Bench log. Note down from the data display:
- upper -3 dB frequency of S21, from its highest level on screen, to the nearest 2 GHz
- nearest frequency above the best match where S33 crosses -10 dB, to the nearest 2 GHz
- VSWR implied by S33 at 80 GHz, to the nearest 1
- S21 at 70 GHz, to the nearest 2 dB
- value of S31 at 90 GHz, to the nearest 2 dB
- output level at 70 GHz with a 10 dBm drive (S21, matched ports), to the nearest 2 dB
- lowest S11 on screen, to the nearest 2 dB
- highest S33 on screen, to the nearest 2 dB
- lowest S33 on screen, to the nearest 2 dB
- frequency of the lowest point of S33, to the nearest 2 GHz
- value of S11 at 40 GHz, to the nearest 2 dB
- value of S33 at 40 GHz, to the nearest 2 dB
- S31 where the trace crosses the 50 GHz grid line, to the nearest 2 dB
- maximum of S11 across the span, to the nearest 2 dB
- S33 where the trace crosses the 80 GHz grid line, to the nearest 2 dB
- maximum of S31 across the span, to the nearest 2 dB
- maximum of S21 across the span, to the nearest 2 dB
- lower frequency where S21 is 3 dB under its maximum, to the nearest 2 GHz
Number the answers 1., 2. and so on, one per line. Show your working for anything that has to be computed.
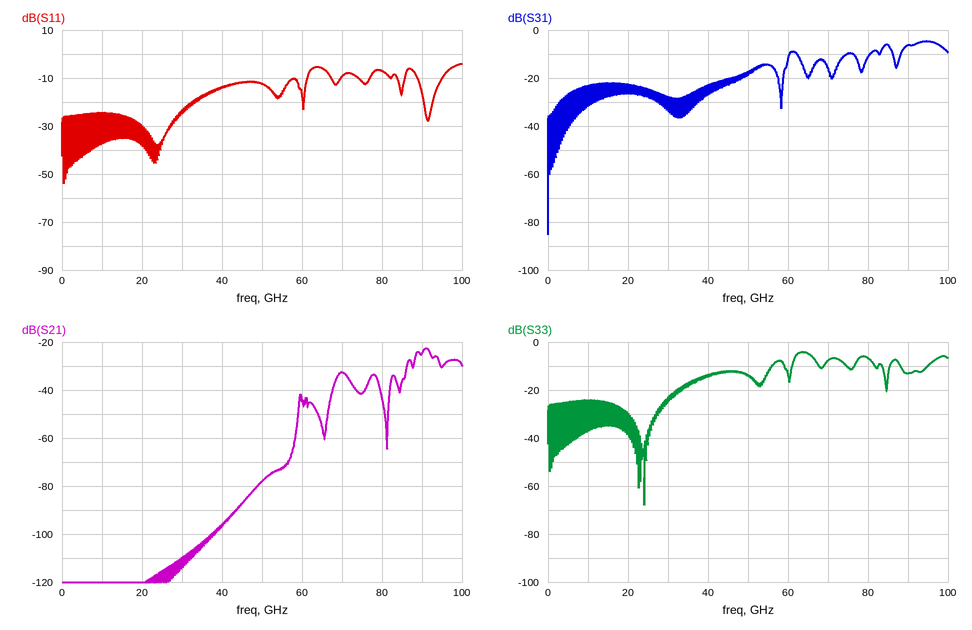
1. 92 GHz
2. 56 GHz
3. |Γ| = 10^(-6/20) = 0.5012; VSWR = (1 + 0.5012)/(1 − 0.5012) ≈ 3
4. -32 dB
5. -6 dB
6. 10 dBm + (-32 dB) = -22 dBm
7. -54 dB
8. -4 dB
9. -68 dB
10. 24 GHz
11. -14 dB
12. -14 dB
13. -18 dB
14. -4 dB
15. -6 dB
16. -4 dB
17. -22 dB
18. 88 GHz
